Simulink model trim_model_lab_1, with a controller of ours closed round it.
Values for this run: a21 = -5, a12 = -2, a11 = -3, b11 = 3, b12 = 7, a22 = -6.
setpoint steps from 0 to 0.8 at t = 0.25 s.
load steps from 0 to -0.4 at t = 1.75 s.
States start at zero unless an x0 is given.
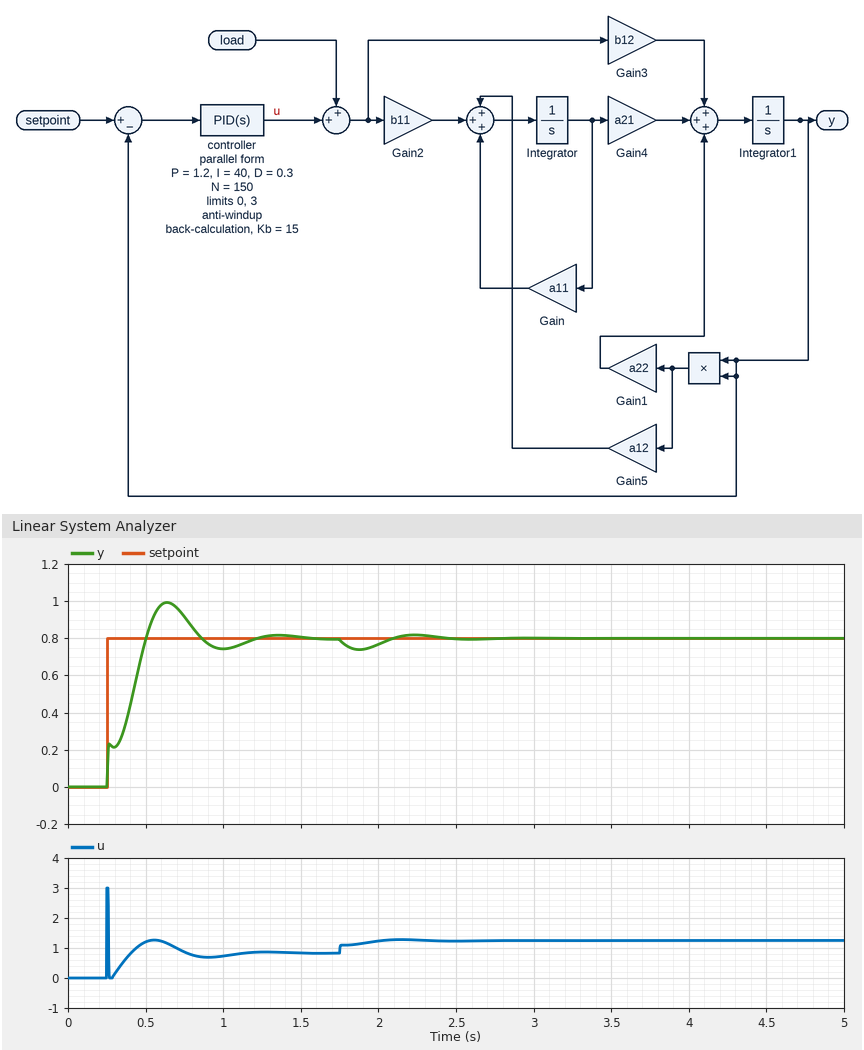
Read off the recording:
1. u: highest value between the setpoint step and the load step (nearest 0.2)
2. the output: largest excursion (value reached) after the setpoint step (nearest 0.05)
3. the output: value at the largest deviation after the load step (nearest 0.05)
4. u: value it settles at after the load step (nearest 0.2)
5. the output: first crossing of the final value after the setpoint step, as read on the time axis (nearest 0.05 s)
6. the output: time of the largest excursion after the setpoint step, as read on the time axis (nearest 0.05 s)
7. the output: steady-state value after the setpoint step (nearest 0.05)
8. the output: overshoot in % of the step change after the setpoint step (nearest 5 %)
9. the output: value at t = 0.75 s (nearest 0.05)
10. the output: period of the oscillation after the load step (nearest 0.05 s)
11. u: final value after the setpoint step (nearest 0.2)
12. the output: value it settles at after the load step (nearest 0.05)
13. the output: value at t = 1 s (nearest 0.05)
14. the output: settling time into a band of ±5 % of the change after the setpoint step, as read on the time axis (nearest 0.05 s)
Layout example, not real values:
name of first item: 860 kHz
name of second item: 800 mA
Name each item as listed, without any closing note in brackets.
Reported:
u: highest value between the setpoint step and the load step: 3.0
the output: largest excursion (value reached) after the setpoint step: 1.00
the output: value at the largest deviation after the load step: 0.75
u: value it settles at after the load step: 1.2
the output: first crossing of the final value after the setpoint step, as read on the time axis: 0.50 s
the output: time of the largest excursion after the setpoint step, as read on the time axis: 0.65 s
the output: steady-state value after the setpoint step: 0.80
the output: overshoot in % of the step change after the setpoint step: 25 %
the output: value at t = 0.75 s: 0.90
the output: period of the oscillation after the load step: 0.70 s
u: final value after the setpoint step: 0.8
the output: value it settles at after the load step: 0.80
the output: value at t = 1 s: 0.75
the output: settling time into a band of ±5 % of the change after the setpoint step, as read on the time axis: 1.10 s
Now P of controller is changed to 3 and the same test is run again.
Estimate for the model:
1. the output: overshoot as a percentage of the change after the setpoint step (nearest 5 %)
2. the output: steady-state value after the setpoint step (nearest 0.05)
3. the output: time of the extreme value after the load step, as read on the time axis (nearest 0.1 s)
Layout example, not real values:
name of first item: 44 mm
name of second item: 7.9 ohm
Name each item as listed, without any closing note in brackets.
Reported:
the output: overshoot as a percentage of the change after the setpoint step: 10 %
the output: steady-state value after the setpoint step: 0.80
the output: time of the extreme value after the load step, as read on the time axis: 1.9 s
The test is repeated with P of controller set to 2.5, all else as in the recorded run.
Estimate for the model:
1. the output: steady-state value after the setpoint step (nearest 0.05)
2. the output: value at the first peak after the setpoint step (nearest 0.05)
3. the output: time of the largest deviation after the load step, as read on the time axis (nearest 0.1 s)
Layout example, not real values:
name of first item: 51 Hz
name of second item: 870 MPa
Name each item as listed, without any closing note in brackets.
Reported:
the output: steady-state value after the setpoint step: 0.80
the output: value at the first peak after the setpoint step: 0.90
the output: time of the largest deviation after the load step, as read on the time axis: 1.9 s
